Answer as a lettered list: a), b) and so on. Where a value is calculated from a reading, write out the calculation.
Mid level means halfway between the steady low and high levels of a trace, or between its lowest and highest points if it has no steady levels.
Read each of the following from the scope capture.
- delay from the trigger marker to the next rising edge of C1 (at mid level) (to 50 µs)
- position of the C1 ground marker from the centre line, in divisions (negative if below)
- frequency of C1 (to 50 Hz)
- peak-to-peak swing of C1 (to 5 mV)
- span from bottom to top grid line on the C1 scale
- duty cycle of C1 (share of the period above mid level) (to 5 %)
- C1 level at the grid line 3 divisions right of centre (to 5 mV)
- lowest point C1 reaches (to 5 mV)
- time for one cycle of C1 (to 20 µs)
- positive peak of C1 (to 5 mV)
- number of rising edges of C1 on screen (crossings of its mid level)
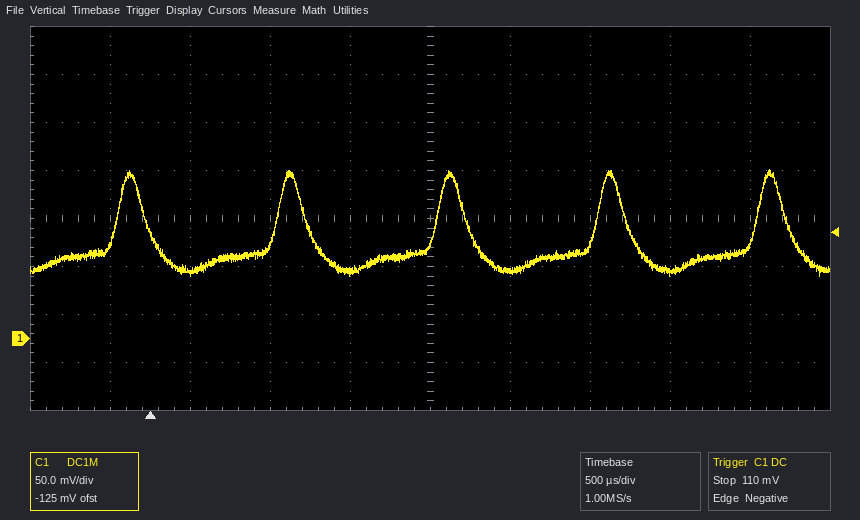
a) 800 µs
b) -2.5 div
c) 1 / 1.00 ms ≈ 1.00 kHz
d) 175 mV − (65 mV) = 110 mV
e) 400 mV
f) 20 %
g) 70 mV
h) 65 mV
i) 1.00 ms
j) 175 mV
k) 5
